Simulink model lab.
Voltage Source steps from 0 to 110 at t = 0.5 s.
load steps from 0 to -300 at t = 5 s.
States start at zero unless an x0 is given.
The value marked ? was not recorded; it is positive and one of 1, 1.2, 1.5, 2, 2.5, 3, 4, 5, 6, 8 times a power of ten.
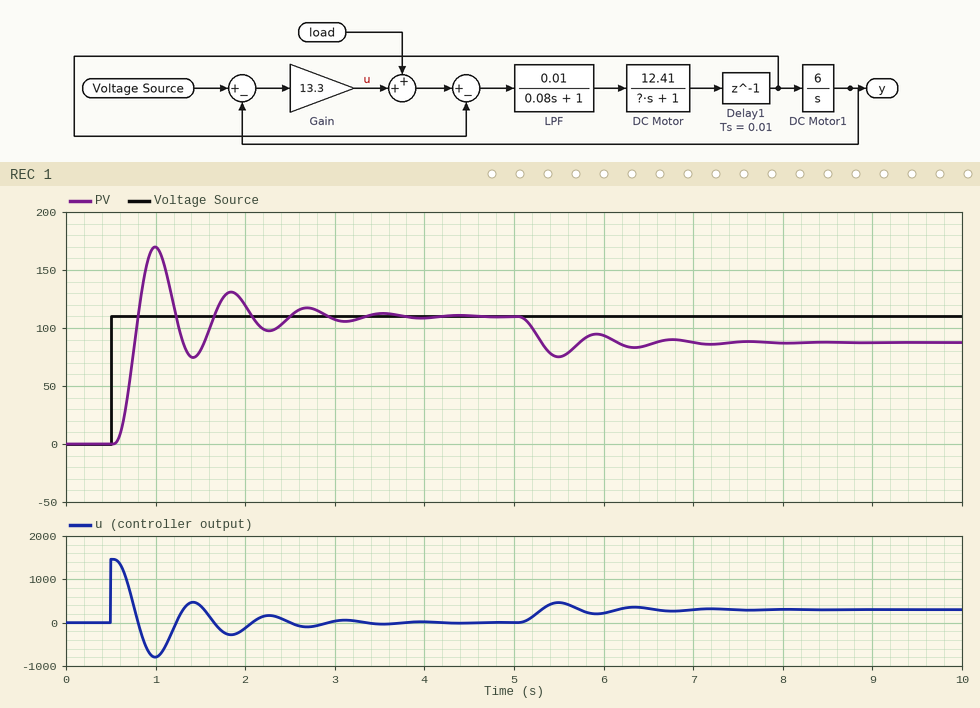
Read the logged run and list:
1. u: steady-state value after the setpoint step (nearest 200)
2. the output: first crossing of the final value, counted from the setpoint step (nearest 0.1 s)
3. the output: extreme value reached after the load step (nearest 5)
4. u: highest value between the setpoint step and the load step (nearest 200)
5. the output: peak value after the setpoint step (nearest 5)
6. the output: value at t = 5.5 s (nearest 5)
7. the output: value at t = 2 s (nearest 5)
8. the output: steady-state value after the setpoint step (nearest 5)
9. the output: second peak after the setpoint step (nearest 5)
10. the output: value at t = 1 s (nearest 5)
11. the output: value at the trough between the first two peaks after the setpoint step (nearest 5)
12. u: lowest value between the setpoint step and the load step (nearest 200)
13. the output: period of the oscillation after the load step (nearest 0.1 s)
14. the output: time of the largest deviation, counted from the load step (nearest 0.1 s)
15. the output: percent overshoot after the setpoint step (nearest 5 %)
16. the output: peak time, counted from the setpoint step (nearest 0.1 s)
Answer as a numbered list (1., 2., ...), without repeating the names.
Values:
1. 0
2. 0.3 s
3. 75
4. 1400
5. 170
6. 75
7. 120
8. 110
9. 130
10. 170
11. 75
12. -800
13. 0.8 s
14. 0.5 s
15. 55 %
16. 0.5 s
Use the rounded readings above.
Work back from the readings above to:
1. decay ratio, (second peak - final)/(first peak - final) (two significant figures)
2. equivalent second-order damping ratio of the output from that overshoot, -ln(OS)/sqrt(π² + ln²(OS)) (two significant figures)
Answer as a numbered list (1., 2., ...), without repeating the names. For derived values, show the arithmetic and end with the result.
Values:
1. (130 - 110) / (170 - 110) = 0.33
2. ln(0.55) = -0.598; 0.598 / sqrt(9.870 + 0.357) = 0.19
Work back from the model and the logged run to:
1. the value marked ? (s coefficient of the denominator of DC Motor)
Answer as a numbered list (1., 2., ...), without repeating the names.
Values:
1. 0.12
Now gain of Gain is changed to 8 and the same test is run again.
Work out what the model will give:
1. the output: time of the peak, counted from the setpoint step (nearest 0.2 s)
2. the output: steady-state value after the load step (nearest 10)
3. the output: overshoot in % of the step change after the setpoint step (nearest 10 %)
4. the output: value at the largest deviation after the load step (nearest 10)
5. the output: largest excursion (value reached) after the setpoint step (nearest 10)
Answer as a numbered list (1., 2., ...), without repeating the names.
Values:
1. 0.6 s
2. 70
3. 30 %
4. 60
5. 140
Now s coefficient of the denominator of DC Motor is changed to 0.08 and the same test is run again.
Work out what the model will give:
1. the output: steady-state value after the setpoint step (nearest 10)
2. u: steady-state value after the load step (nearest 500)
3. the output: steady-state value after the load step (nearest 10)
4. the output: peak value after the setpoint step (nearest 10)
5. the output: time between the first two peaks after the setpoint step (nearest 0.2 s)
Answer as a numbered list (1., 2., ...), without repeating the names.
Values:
1. 110
2. 500
3. 90
4. 160
5. 0.8 s
